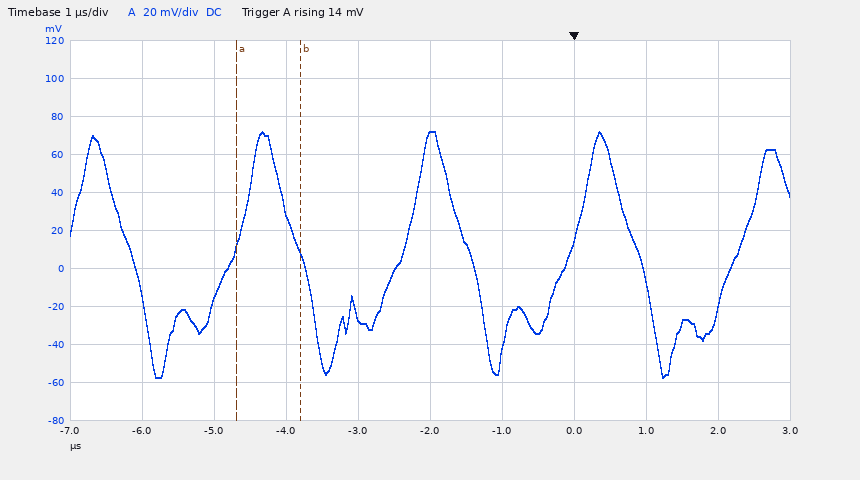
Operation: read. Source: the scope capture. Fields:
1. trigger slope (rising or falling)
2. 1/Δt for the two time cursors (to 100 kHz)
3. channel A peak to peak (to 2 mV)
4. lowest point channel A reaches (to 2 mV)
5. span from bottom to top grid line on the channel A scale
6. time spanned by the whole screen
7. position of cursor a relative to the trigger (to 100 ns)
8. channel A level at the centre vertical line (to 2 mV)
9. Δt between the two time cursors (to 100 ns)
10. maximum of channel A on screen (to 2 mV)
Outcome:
rising
1.1 MHz
130 mV
-58 mV
200 mV
10 µs
-4.7 µs
70 mV
900 ns
72 mV
